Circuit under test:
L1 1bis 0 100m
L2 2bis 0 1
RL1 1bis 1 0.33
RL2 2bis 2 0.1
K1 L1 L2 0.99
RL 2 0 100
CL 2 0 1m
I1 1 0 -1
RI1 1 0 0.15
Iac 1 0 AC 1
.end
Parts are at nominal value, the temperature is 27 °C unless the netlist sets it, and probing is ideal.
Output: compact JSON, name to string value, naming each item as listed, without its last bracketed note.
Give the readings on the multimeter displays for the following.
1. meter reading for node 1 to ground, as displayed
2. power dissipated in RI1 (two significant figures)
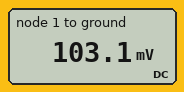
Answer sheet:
{"meter reading for node 1 to ground, as displayed": "103.1 mV", "power dissipated in RI1": "71 mW"}
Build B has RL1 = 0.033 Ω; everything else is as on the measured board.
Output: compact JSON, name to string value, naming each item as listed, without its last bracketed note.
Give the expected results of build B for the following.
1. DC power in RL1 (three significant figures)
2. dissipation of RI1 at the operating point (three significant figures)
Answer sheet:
{"DC power in RL1": "22.2 mW", "dissipation of RI1 at the operating point": "4.88 mW"}
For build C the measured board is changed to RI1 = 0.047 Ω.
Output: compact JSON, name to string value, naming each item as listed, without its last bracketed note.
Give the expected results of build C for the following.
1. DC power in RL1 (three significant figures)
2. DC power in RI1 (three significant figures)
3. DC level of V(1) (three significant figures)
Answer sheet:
{"DC power in RL1": "5.13 mW", "DC power in RI1": "36.0 mW", "DC level of V(1)": "41.1 mV"}
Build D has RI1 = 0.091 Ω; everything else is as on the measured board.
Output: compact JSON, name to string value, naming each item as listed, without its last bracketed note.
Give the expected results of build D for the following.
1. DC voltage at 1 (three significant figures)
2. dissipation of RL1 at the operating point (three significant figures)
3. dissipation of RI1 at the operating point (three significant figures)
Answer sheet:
{"DC voltage at 1": "71.3 mV", "dissipation of RL1 at the operating point": "15.4 mW", "dissipation of RI1 at the operating point": "55.9 mW"}
